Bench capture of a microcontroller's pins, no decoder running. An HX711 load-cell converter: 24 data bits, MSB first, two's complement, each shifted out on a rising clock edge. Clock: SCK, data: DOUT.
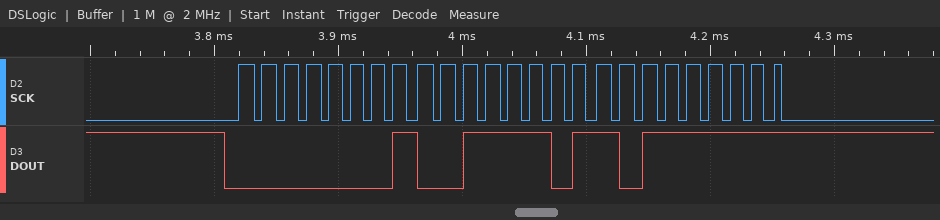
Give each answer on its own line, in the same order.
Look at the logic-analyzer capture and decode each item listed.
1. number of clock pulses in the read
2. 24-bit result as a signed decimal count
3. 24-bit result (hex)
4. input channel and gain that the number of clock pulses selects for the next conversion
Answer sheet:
25
81343
0x013DBF
channel A, gain 128
